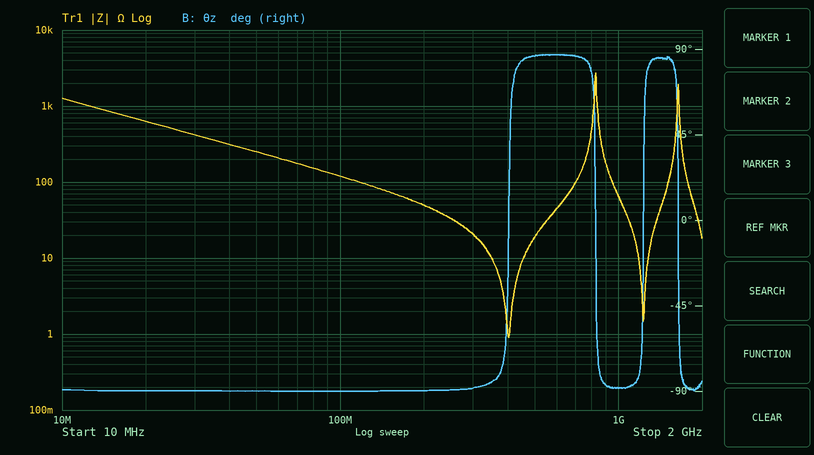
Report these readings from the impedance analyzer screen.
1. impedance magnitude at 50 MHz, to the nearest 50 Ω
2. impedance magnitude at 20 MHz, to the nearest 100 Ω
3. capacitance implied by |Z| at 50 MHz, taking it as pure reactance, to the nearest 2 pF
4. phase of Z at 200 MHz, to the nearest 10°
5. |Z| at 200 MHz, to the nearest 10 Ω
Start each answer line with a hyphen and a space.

- 250 Ω
- 600 Ω
- 12 pF
- -90°
- 50 Ω
